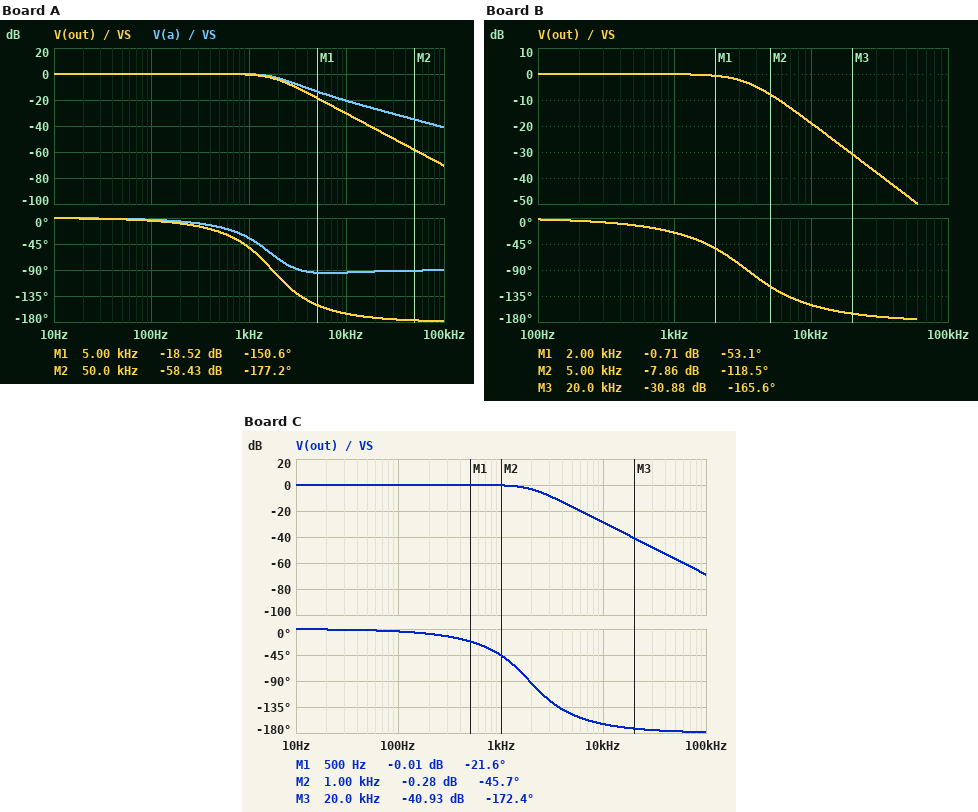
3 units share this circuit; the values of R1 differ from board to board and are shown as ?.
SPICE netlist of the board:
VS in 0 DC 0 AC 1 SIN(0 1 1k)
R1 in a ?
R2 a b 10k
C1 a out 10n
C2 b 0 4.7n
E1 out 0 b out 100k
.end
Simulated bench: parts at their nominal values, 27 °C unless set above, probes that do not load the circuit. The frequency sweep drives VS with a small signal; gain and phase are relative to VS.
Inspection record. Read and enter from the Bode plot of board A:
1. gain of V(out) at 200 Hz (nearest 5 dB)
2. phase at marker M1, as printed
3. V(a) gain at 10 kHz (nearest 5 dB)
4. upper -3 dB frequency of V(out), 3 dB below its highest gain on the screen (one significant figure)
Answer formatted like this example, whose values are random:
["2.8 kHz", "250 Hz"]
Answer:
["0 dB", "-150.6 deg", "-20 dB", "2 kHz"]
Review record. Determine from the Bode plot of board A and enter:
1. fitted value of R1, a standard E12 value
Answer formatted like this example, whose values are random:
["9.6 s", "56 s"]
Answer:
["18 kΩ"]
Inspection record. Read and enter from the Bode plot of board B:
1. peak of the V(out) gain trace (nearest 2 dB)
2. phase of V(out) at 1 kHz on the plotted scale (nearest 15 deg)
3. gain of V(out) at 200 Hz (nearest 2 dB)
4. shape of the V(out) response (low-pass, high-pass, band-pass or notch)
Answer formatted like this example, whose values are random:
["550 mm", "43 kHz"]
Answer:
["0 dB", "-30 deg", "0 dB", "low-pass"]
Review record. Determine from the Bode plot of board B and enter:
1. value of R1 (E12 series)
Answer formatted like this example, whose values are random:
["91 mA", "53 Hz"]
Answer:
["4.7 kΩ"]
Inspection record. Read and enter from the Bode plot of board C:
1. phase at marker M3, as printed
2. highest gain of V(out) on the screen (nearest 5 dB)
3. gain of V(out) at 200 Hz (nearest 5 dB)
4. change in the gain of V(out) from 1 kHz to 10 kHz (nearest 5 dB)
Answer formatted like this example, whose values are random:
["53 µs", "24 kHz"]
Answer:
["-172.4 deg", "0 dB", "0 dB", "-30 dB"]
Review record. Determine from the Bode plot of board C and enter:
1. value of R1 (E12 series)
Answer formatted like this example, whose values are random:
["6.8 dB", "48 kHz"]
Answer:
["15 kΩ"]
